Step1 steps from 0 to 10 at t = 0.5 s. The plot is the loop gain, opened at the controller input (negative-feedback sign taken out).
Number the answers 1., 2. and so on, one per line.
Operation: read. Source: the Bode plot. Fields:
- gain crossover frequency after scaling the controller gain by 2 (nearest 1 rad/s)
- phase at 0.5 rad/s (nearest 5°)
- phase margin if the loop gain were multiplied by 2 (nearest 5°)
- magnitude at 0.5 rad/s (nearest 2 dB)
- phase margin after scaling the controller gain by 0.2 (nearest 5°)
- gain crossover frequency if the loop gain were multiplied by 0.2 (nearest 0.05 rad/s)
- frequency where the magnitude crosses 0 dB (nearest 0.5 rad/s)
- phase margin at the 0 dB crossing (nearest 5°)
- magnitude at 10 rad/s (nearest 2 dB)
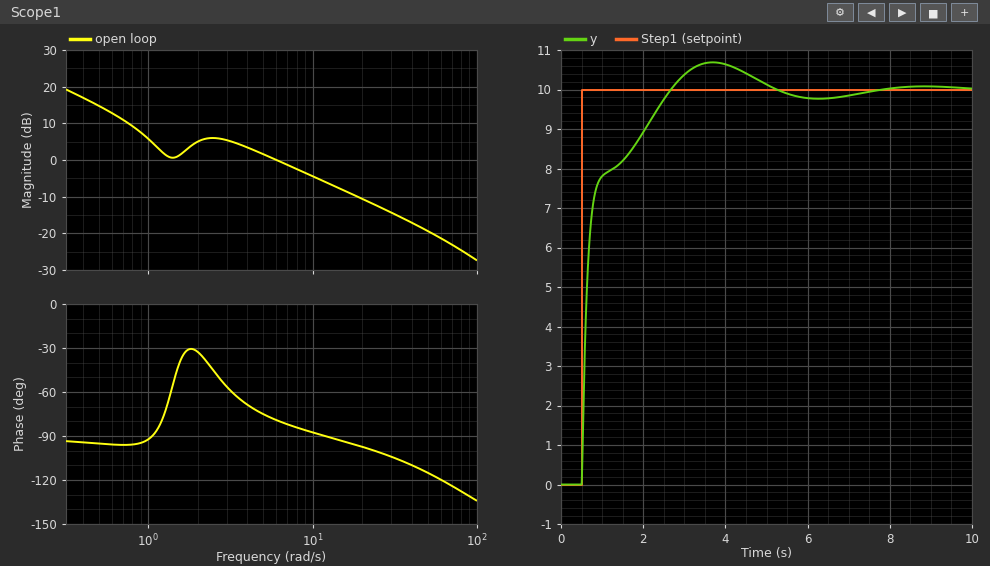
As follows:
1. 12 rad/s
2. -95°
3. 90°
4. 14 dB
5. 85°
6. 0.55 rad/s
7. 6.0 rad/s
8. 100°
9. -4 dB
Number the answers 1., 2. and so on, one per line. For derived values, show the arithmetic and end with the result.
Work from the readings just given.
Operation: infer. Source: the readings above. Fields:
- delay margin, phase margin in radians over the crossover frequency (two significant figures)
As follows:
1. 100 × π / 180 / 6 = 0.29 s
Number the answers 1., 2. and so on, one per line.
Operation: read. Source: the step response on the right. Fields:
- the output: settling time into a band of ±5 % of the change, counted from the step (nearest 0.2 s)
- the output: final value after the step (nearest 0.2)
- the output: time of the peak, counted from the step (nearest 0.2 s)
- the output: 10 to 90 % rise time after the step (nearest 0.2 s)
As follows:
1. 3.8 s
2. 10.0
3. 3.2 s
4. 1.6 s
